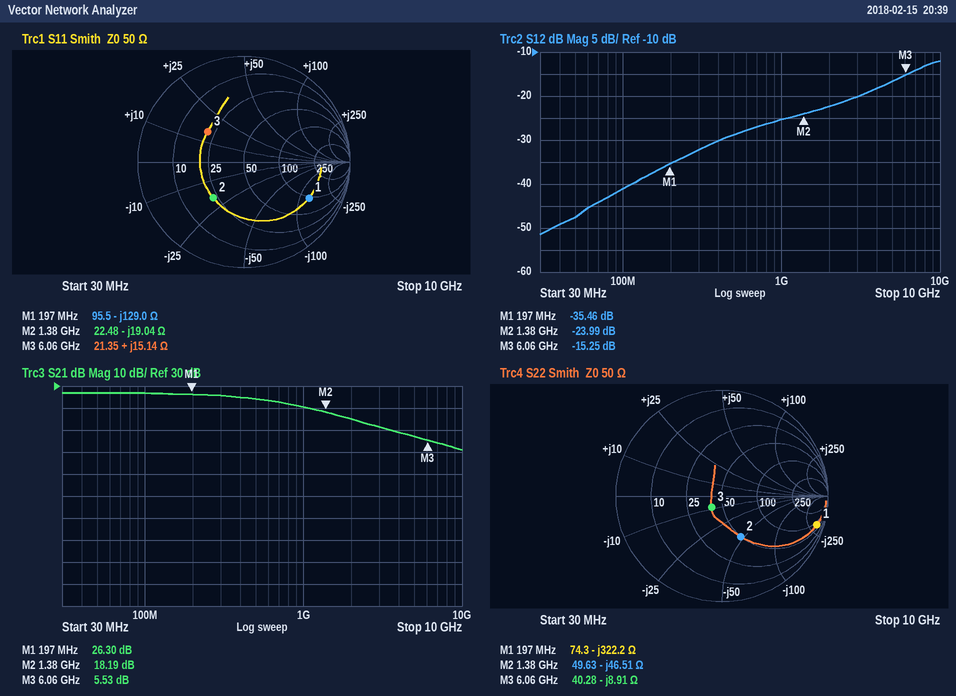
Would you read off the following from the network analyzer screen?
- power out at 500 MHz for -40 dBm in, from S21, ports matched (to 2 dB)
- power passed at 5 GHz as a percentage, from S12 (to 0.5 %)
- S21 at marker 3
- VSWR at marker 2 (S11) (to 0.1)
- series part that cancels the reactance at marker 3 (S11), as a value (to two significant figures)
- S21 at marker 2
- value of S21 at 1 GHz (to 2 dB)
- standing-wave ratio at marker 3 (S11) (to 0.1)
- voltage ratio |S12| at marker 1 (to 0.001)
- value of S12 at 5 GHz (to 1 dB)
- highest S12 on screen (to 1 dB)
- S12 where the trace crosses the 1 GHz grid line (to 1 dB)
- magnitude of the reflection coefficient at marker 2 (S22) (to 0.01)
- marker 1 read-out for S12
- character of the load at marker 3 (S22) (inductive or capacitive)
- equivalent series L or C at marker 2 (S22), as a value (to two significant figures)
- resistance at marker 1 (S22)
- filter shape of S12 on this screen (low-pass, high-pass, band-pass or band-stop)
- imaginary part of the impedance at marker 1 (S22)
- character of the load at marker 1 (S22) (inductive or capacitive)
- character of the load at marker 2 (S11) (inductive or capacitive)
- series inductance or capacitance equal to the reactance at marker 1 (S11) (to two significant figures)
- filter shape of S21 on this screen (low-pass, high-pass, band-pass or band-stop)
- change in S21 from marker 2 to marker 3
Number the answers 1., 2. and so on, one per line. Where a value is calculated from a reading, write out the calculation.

1. -40 dBm + (24 dB) = -16 dBm
2. 10^(-17/10) ≈ 2.0 %
3. 5.53 dB
4. 2.6
5. C = 1/(2π × 6.06 GHz × 15.14 Ω) ≈ 1.7 pF
6. 18.19 dB
7. 20 dB
8. 2.6
9. 10^(-35.46/20) ≈ 0.017
10. -17 dB
11. -12 dB
12. -25 dB
13. 0.42
14. -35.46 dB
15. capacitive
16. C = 1/(2π × 1.38 GHz × 46.51 Ω) ≈ 2.5 pF
17. 74.3 Ω
18. high-pass
19. -322.2 Ω
20. capacitive
21. capacitive
22. C = 1/(2π × 197 MHz × 129 Ω) ≈ 6.3 pF
23. low-pass
24. 5.53 − (18.19) = -12.66 dB
